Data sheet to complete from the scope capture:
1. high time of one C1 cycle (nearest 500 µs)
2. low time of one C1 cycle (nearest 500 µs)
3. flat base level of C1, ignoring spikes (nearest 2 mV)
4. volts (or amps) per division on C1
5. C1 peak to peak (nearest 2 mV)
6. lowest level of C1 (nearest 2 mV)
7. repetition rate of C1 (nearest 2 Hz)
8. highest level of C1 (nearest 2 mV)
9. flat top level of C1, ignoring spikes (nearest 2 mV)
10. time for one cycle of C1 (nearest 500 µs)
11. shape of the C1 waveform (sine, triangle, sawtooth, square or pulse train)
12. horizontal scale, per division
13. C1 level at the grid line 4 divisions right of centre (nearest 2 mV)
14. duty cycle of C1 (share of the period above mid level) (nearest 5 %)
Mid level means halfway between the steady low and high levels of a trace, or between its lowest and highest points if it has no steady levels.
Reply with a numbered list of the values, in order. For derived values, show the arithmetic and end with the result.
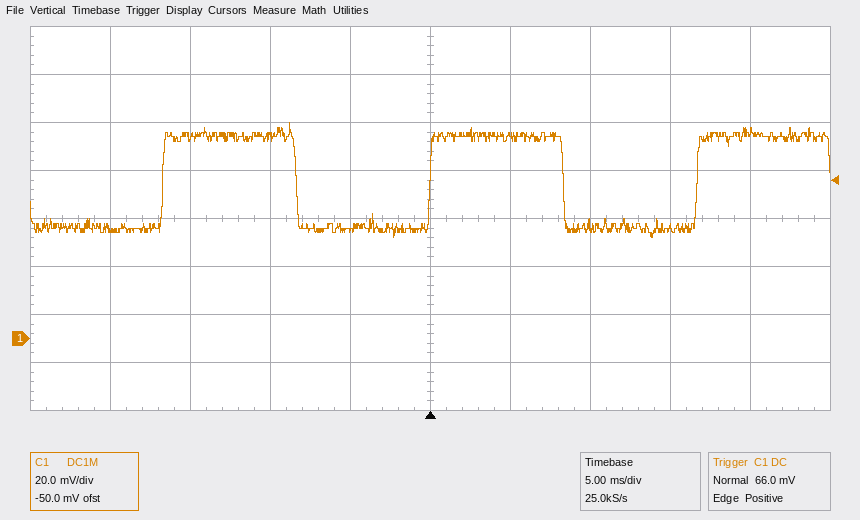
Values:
1. 8.5 ms
2. 8.5 ms
3. 46 mV
4. 20 mV
5. 90 mV − (42 mV) = 48 mV
6. 42 mV
7. 1 / 16.5 ms ≈ 60.6 Hz, so 60 Hz to the nearest 2 Hz
8. 90 mV
9. 84 mV
10. 16.5 ms
11. square
12. 5 ms
13. 86 mV
14. 8.5 ms / 16.5 ms ≈ 51.5 %, so 50 % to the nearest 5 %
